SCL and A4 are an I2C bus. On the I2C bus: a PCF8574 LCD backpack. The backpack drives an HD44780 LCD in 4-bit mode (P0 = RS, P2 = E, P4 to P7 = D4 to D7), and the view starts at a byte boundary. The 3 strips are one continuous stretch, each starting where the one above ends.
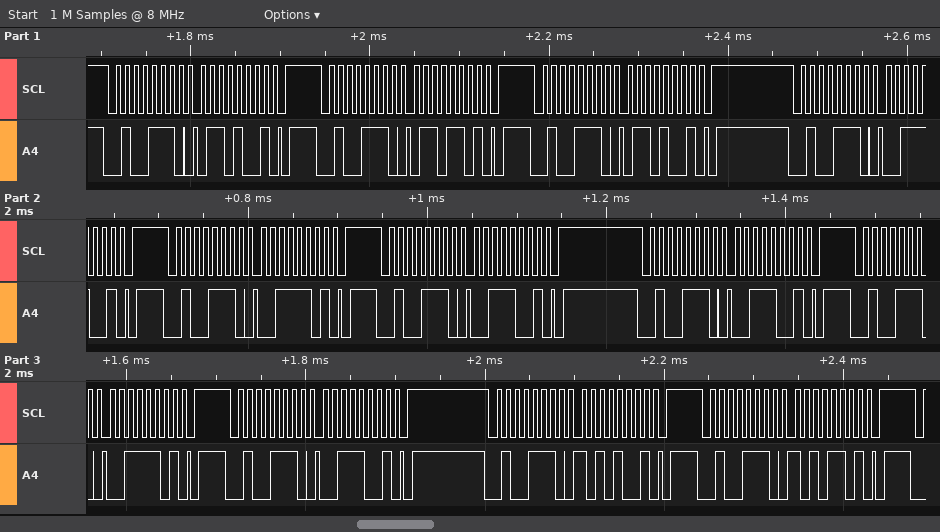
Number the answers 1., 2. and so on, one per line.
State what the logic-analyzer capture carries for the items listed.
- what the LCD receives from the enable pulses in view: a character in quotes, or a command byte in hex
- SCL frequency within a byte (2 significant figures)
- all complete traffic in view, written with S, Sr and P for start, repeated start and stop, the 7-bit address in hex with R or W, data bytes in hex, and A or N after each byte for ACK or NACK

1. 'c'
2. 100 kHz
3. S 27W A 69 A P S 27W A 6D A P S 27W A 69 A P S 27W A 39 A P S 27W A 3D A P S 27W A 39 A P S 27W A 39 A P S 27W A 3D A P S 27W A 39 A P S 27W A A9 A P S 27W A AD A P
